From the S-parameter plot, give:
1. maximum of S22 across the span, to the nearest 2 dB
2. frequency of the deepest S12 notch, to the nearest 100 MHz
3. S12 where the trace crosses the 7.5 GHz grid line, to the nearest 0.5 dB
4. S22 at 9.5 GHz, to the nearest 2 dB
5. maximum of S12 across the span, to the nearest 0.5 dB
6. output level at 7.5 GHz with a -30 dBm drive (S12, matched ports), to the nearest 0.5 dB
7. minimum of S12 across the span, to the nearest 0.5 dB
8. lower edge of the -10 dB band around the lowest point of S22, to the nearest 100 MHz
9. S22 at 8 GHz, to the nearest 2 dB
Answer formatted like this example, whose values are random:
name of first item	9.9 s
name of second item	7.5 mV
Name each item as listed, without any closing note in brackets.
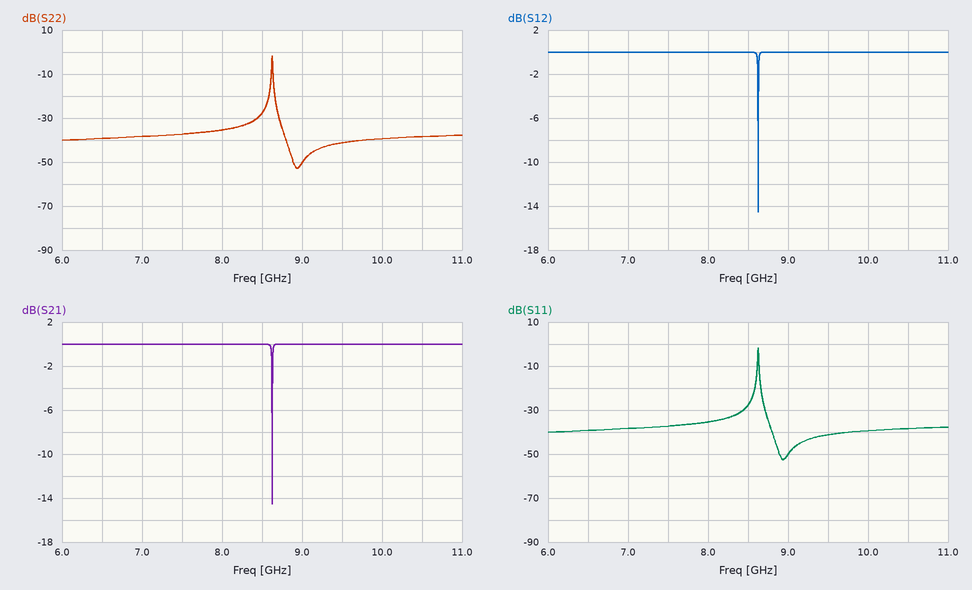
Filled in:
maximum of S22 across the span, to the nearest 2 dB	-2 dB
frequency of the deepest S12 notch, to the nearest 100 MHz	8.6 GHz
S12 where the trace crosses the 7.5 GHz grid line, to the nearest 0.5 dB	0.0 dB
S22 at 9.5 GHz, to the nearest 2 dB	-42 dB
maximum of S12 across the span, to the nearest 0.5 dB	0.0 dB
output level at 7.5 GHz with a -30 dBm drive (S12, matched ports), to the nearest 0.5 dB	-30.0 dBm
minimum of S12 across the span, to the nearest 0.5 dB	-14.5 dB
lower edge of the -10 dB band around the lowest point of S22, to the nearest 100 MHz	8.6 GHz
S22 at 8 GHz, to the nearest 2 dB	-36 dB
